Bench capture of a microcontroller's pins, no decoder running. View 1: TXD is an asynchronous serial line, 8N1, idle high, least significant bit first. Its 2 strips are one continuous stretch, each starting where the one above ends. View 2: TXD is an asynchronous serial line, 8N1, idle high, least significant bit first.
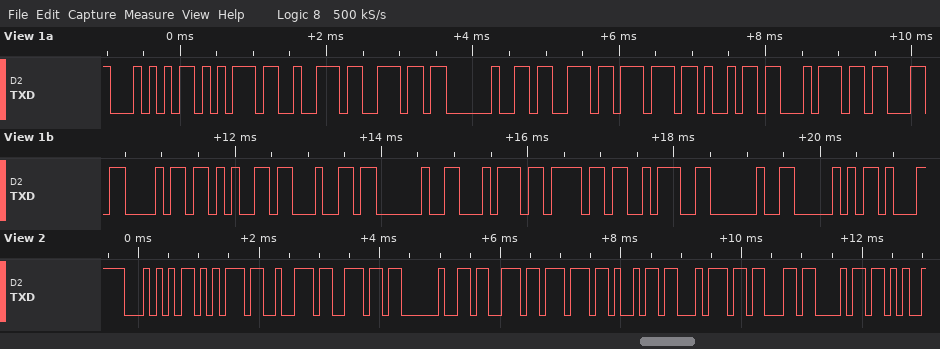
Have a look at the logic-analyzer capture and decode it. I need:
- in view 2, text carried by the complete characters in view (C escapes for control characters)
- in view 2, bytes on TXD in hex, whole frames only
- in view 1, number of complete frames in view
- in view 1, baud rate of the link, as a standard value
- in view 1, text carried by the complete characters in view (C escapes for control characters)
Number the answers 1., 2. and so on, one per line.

1. "Turn switch"
2. 54 75 72 6E 20 73 77 69 74 63 68
3. 19
4. 9600 baud
5. "Turn switched to: P"
